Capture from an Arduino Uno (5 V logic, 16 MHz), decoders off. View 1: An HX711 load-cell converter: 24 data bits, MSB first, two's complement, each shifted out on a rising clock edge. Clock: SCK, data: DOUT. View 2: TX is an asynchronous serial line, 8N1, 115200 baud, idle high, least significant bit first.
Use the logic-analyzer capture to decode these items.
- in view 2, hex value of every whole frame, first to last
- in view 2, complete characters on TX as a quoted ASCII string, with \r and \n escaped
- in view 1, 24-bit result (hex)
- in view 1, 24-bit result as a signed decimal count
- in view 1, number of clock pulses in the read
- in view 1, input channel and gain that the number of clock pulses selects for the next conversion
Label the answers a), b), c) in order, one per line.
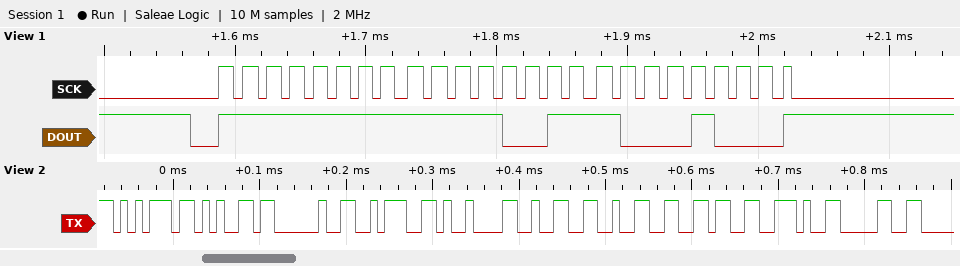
a) 0x75 0x65 0x20 0x3A 0x09 0x32 0x32 0x36 0x2E 0x30
b) "ue :\t226.0"
c) 0xFFF388
d) -3192
e) 25
f) channel A, gain 128
